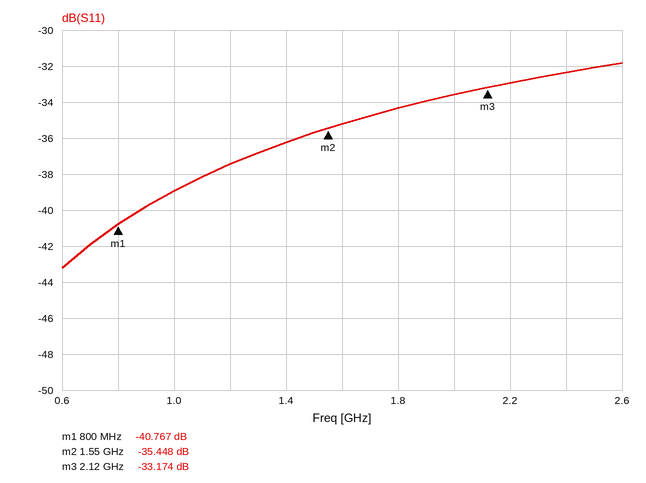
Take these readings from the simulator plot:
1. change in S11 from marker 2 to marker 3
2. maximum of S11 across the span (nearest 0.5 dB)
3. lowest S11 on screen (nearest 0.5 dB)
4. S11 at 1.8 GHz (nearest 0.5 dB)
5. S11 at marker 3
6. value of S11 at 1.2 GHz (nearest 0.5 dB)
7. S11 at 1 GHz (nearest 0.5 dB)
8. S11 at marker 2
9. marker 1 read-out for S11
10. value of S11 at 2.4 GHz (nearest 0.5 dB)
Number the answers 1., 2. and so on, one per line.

1. 2.274 dB
2. -32.0 dB
3. -43.0 dB
4. -34.5 dB
5. -33.174 dB
6. -37.5 dB
7. -39.0 dB
8. -35.448 dB
9. -40.767 dB
10. -32.5 dB
